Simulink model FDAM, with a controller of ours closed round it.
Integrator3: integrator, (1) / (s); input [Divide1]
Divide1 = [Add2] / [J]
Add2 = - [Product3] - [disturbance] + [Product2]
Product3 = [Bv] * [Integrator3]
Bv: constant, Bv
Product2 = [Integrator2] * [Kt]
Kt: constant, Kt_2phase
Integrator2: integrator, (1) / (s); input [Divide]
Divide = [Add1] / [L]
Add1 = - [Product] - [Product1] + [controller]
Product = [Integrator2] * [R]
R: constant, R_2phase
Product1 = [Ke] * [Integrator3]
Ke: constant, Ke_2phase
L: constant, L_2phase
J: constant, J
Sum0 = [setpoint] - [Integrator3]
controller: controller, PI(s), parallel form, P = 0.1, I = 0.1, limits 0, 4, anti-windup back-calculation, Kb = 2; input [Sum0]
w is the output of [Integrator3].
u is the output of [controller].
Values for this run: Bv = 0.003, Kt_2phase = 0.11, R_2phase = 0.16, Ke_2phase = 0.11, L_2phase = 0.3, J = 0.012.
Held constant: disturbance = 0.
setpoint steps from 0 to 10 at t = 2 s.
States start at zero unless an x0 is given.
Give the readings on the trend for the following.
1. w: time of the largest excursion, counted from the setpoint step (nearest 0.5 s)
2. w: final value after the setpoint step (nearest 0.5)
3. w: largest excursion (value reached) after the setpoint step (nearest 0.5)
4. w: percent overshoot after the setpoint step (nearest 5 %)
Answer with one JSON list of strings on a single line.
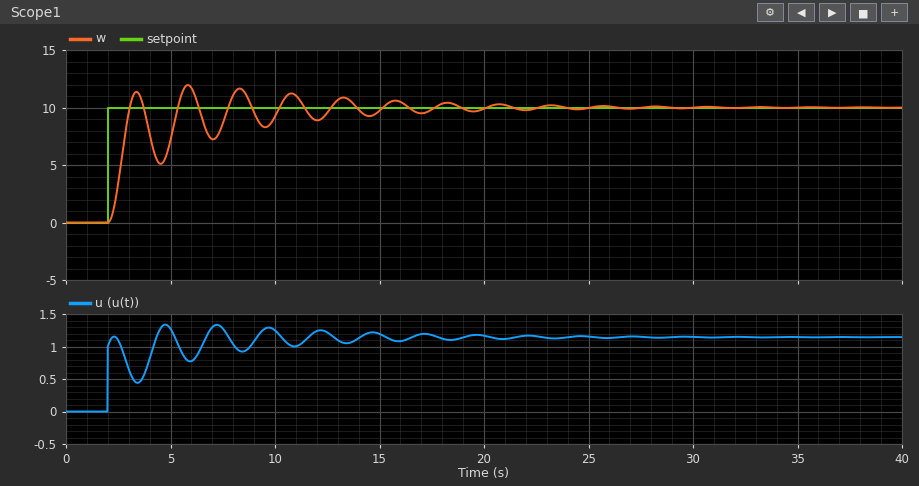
["4.0 s", "10.0", "12.0", "20 %"]
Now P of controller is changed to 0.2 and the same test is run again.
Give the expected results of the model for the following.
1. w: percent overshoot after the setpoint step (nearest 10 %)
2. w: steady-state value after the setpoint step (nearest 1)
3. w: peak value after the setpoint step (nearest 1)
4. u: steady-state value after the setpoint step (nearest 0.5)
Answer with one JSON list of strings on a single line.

["30 %", "10", "13", "1.0"]
